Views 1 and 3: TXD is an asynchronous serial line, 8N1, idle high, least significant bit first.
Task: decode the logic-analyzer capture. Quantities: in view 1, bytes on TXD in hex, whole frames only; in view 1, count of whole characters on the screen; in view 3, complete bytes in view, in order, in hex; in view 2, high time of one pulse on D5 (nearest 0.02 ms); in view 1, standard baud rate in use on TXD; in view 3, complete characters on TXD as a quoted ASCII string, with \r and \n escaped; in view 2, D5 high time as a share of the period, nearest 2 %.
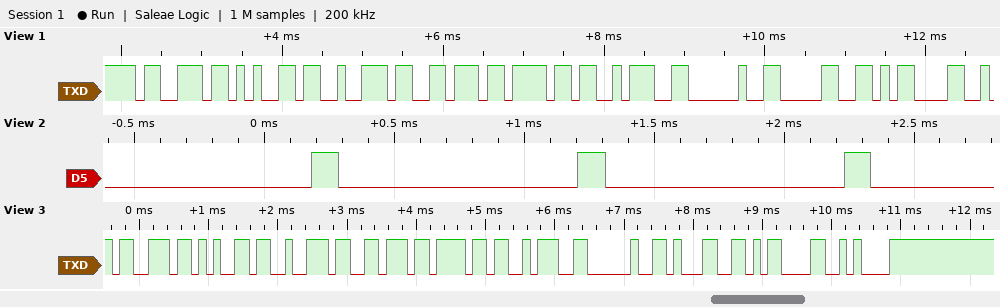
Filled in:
73 65 72 76 6F 3A 20 30 0D
9
73 65 72 76 6F 3A 20 31 0D 0A
0.10 ms
9600 baud
"servo: 1\r\n"
10 %
